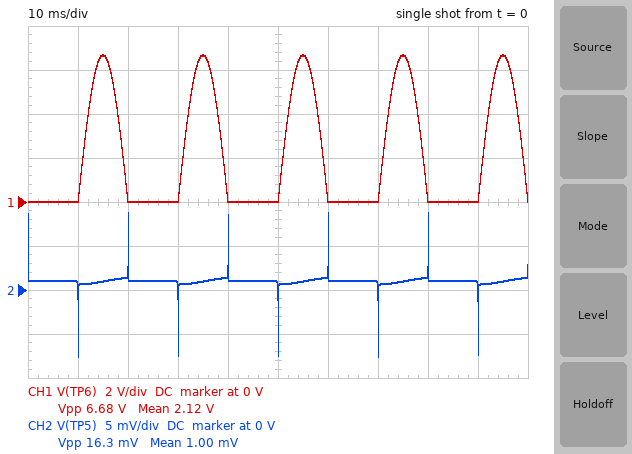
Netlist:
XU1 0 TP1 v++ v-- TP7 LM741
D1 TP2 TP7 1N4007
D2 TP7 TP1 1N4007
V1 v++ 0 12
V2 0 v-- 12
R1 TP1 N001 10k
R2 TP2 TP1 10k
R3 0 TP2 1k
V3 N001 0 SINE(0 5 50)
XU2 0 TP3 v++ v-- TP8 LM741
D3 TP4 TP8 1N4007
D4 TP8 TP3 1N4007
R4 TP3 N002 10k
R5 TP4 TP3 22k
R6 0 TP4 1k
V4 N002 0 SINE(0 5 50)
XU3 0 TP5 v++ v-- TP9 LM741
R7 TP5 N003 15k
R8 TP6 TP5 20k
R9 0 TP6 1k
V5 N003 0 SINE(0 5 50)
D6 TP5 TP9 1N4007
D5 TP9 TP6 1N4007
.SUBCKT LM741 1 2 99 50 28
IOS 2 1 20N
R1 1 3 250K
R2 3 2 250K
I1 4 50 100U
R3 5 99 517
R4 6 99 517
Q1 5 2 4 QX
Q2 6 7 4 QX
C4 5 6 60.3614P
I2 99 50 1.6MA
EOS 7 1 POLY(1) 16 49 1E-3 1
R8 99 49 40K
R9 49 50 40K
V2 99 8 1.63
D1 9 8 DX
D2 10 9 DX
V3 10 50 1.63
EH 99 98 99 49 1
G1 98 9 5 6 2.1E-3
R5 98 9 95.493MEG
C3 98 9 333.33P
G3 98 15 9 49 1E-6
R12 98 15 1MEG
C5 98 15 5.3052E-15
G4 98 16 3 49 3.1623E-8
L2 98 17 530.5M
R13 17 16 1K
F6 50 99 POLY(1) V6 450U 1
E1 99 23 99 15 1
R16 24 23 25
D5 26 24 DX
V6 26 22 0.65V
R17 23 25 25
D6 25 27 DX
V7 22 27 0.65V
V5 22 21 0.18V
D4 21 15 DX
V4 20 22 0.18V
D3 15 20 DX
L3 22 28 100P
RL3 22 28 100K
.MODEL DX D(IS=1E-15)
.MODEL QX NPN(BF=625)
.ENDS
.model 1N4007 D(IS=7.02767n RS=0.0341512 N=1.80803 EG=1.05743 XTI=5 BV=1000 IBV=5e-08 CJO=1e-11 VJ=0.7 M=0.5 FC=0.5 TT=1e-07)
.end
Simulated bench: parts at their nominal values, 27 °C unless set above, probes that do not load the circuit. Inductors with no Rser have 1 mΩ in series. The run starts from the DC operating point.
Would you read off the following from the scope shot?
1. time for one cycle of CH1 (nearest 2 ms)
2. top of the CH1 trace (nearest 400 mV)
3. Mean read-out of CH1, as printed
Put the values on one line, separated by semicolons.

20 ms; 6.8 V; 2.12 V
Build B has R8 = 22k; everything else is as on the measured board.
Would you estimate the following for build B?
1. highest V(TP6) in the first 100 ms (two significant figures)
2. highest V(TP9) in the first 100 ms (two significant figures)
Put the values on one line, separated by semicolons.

7.3 V; 8.0 V
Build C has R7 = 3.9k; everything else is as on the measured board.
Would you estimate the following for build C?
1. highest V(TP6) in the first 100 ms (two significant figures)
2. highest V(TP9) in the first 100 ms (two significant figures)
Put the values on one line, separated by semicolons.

10 V; 11 V
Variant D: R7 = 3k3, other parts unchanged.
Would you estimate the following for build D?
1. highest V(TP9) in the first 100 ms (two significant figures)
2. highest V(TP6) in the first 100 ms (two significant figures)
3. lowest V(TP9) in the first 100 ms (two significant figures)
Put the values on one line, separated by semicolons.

11 V; 10 V; -570 mV
